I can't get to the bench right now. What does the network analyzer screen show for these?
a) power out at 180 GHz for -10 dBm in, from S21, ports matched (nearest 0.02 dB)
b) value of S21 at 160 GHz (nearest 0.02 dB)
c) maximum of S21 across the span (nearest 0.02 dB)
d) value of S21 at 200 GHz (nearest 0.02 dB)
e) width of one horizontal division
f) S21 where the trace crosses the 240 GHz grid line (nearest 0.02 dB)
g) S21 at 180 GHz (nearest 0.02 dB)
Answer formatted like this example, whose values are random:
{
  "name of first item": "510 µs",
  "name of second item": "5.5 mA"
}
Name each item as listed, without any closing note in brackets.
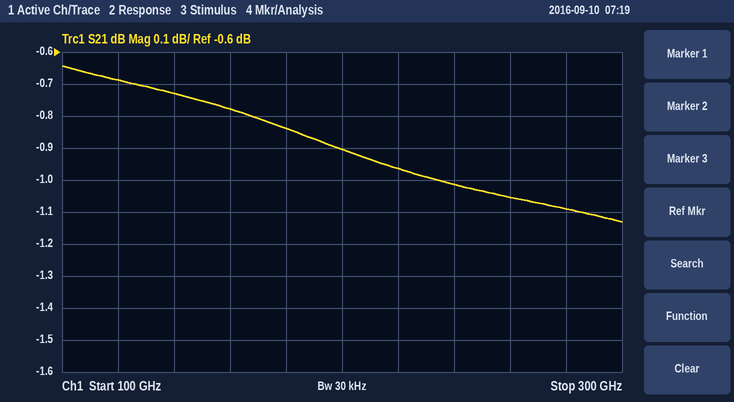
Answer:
{
  "power out at 180 GHz for -10 dBm in, from S21, ports matched": "-10.84 dBm",
  "value of S21 at 160 GHz": "-0.78 dB",
  "maximum of S21 across the span": "-0.64 dB",
  "value of S21 at 200 GHz": "-0.90 dB",
  "width of one horizontal division": "20 GHz",
  "S21 where the trace crosses the 240 GHz grid line": "-1.02 dB",
  "S21 at 180 GHz": "-0.84 dB"
}
